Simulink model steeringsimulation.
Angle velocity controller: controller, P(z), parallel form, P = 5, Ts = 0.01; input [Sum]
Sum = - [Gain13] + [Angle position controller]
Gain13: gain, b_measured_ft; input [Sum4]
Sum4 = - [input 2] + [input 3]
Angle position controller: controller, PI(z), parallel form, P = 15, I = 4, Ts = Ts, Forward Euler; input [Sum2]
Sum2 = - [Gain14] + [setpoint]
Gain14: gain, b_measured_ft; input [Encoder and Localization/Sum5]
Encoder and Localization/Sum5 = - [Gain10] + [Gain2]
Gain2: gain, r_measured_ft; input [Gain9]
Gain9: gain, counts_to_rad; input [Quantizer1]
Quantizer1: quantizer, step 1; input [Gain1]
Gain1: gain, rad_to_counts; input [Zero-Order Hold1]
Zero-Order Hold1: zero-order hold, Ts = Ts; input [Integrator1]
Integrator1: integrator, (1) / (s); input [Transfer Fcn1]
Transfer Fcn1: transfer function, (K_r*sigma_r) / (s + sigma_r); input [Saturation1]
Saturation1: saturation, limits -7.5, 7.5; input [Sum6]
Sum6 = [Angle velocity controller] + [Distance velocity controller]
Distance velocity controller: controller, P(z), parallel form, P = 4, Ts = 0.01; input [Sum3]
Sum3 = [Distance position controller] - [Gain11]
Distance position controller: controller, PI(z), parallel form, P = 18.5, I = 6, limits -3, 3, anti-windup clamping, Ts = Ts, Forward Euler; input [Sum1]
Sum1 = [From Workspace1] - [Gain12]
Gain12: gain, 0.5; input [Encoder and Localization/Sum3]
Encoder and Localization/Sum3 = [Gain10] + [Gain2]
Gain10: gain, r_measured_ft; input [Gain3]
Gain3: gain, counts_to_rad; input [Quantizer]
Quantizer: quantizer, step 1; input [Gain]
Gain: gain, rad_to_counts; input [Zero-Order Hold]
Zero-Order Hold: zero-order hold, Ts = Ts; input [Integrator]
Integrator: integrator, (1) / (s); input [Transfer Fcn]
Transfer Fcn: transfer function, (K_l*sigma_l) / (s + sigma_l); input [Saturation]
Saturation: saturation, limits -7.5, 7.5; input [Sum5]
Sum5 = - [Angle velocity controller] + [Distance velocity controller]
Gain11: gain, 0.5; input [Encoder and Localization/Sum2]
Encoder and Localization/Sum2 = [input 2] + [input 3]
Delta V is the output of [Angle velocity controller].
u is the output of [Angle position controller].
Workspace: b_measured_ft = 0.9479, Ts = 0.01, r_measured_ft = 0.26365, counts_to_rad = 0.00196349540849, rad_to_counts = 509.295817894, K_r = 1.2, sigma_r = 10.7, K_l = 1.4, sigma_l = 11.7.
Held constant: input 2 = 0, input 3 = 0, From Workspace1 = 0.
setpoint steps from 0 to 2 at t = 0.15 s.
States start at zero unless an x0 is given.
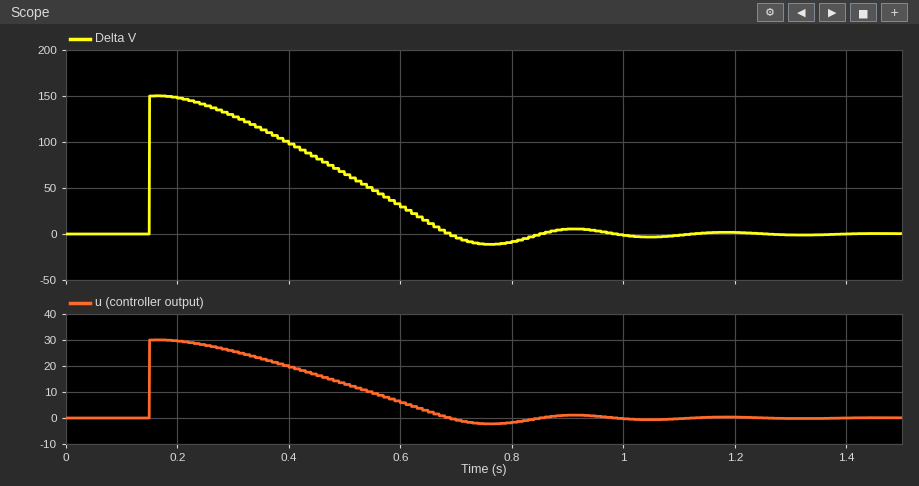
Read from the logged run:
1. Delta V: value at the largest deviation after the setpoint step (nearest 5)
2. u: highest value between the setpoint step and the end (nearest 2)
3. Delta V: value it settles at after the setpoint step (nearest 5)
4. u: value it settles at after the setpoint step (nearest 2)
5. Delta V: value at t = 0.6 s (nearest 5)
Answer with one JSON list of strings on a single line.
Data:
["150", "30", "0", "0", "30"]
